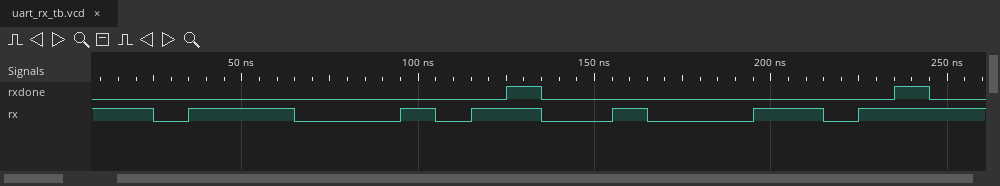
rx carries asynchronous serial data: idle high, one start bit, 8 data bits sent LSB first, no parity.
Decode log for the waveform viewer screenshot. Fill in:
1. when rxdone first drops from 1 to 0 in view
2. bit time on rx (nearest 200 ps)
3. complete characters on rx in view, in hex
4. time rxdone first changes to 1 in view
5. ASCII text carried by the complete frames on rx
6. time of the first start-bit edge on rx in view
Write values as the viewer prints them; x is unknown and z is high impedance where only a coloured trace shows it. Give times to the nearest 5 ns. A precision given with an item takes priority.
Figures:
135 ns
10000 ps
47, 62
125 ns
"Gb"
25 ns
